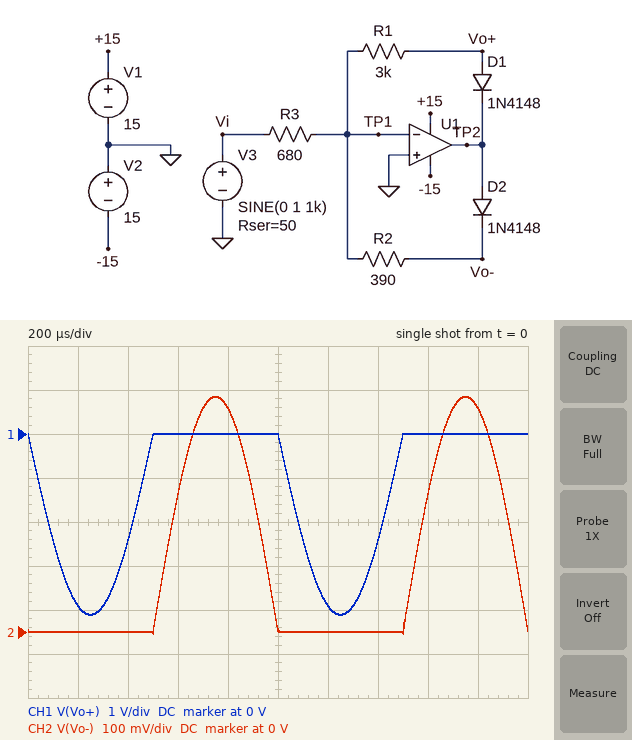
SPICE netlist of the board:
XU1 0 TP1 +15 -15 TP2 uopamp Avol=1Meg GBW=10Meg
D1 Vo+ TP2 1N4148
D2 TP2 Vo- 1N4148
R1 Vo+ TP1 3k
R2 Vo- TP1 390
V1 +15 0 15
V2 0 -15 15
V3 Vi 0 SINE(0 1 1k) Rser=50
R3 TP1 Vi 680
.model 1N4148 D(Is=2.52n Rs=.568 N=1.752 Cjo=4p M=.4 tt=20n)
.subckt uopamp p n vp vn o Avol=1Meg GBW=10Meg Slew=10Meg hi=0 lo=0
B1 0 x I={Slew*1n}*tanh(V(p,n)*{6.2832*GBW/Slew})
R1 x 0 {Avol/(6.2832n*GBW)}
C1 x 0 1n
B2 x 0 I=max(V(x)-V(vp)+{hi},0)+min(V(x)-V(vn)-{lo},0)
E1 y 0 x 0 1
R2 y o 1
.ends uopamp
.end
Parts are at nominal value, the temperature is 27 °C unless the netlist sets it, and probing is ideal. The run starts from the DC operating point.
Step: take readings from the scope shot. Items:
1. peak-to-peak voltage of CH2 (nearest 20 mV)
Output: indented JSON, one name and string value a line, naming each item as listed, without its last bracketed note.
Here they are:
{
  "peak-to-peak voltage of CH2": "540 mV"
}
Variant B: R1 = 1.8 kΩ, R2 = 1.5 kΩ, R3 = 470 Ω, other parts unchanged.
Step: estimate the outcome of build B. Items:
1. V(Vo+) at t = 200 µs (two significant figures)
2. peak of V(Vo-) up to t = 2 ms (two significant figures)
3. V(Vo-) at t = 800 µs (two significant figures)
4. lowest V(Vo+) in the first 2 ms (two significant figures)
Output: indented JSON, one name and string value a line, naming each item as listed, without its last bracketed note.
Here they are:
{
  "V(Vo+) at t = 200 µs": "-3.3 V",
  "peak of V(Vo-) up to t = 2 ms": "2.9 V",
  "V(Vo-) at t = 800 µs": "2.7 V",
  "lowest V(Vo+) in the first 2 ms": "-3.5 V"
}
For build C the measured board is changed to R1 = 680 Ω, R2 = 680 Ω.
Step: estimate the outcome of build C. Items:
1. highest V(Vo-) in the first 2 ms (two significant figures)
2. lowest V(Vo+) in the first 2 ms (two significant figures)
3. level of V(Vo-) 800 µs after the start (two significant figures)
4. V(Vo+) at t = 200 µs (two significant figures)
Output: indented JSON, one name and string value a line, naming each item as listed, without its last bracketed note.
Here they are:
{
  "highest V(Vo-) in the first 2 ms": "930 mV",
  "lowest V(Vo+) in the first 2 ms": "-930 mV",
  "level of V(Vo-) 800 µs after the start": "890 mV",
  "V(Vo+) at t = 200 µs": "-890 mV"
}
